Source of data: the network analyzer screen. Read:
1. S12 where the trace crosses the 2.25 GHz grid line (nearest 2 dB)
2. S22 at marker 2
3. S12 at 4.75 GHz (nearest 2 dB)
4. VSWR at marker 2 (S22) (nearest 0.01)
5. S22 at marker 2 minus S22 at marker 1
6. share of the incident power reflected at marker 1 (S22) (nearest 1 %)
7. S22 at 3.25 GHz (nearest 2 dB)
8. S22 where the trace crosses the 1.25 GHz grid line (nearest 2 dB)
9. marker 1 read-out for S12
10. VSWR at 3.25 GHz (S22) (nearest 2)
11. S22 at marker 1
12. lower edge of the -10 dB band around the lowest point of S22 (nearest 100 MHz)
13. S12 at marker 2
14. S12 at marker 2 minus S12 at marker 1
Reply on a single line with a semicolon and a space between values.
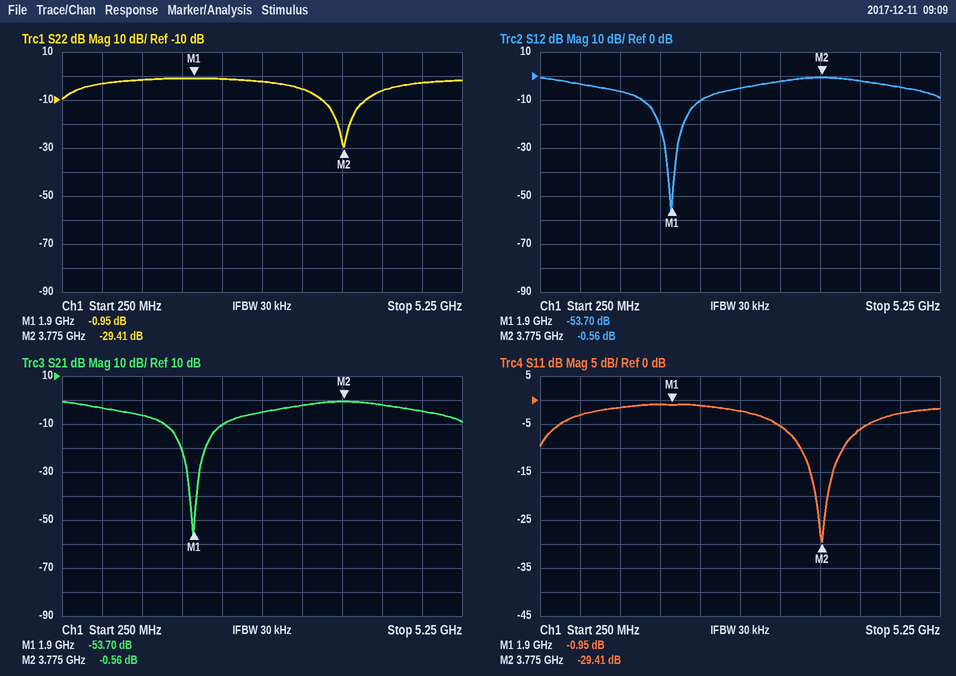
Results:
-10 dB; -29.41 dB; -4 dB; 1.07; -28.46 dB; 80 %; -6 dB; -2 dB; -53.70 dB; 4; -0.95 dB; 3.5 GHz; -0.56 dB; 53.14 dB
